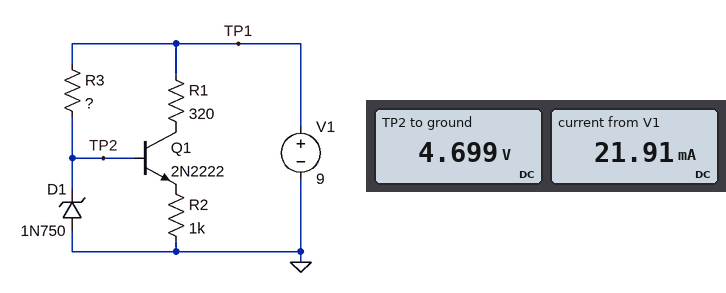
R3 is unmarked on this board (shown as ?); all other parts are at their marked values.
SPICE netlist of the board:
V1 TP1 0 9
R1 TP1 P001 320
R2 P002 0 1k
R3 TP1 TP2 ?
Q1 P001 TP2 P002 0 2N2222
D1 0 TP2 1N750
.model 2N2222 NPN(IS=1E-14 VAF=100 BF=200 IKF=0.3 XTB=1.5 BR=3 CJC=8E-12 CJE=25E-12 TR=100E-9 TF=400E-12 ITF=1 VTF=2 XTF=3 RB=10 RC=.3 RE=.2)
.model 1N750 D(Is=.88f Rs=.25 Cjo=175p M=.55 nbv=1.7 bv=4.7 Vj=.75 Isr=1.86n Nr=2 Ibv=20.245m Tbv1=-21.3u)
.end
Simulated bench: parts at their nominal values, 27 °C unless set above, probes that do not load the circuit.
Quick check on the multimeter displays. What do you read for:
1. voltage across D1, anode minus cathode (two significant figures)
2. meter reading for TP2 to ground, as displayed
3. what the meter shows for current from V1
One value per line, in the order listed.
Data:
-4.7 V
4.699 V
21.91 mA
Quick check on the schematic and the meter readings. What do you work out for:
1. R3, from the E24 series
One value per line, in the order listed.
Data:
240 Ω
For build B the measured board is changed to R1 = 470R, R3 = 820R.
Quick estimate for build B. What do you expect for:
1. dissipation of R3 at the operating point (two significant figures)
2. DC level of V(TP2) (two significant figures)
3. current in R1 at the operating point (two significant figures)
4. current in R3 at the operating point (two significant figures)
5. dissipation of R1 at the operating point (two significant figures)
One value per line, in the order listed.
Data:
23 mW
4.6 V
3.9 mA
5.3 mA
7.3 mW
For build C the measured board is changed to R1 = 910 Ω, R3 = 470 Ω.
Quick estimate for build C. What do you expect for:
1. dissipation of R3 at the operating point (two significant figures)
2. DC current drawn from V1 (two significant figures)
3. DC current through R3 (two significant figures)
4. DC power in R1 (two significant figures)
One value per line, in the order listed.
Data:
40 mW
13 mA
9.2 mA
14 mW
